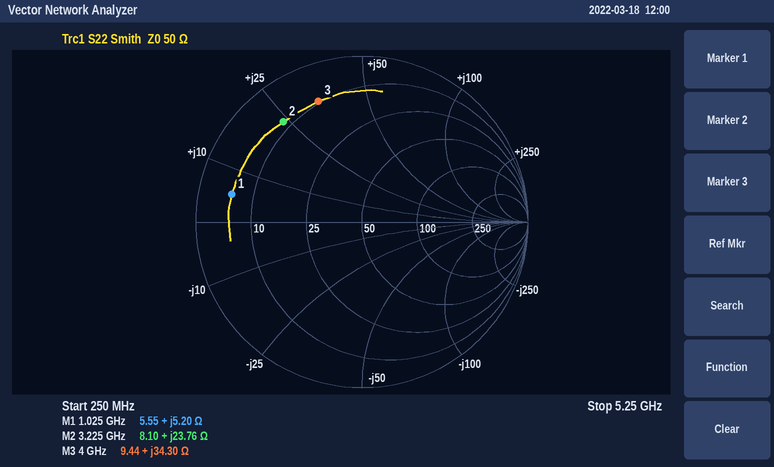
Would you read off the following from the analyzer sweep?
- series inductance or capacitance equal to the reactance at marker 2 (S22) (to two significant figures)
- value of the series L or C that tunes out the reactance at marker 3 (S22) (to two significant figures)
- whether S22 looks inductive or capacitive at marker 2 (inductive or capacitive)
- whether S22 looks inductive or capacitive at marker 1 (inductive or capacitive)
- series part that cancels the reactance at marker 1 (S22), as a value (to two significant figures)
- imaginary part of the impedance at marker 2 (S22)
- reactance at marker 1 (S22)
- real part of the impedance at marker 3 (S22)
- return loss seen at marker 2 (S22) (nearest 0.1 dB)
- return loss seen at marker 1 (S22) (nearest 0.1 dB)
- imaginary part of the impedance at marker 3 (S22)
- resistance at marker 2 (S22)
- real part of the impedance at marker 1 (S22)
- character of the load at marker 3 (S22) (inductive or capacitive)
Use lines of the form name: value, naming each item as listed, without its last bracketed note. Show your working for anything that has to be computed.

series inductance or capacitance equal to the reactance at marker 2 (S22): L = 23.76 Ω/(2π × 3.225 GHz) ≈ 1.2 nH
value of the series L or C that tunes out the reactance at marker 3 (S22): C = 1/(2π × 4 GHz × 34.3 Ω) ≈ 1.2 pF
whether S22 looks inductive or capacitive at marker 2: inductive
whether S22 looks inductive or capacitive at marker 1: inductive
series part that cancels the reactance at marker 1 (S22), as a value: C = 1/(2π × 1.025 GHz × 5.2 Ω) ≈ 30 pF
imaginary part of the impedance at marker 2: +23.76 Ω
reactance at marker 1: +5.20 Ω
real part of the impedance at marker 3: 9.44 Ω
return loss seen at marker 2 (S22): 2.3 dB
return loss seen at marker 1 (S22): 1.9 dB
imaginary part of the impedance at marker 3: +34.30 Ω
resistance at marker 2: 8.10 Ω
real part of the impedance at marker 1: 5.55 Ω
character of the load at marker 3 (S22): inductive
